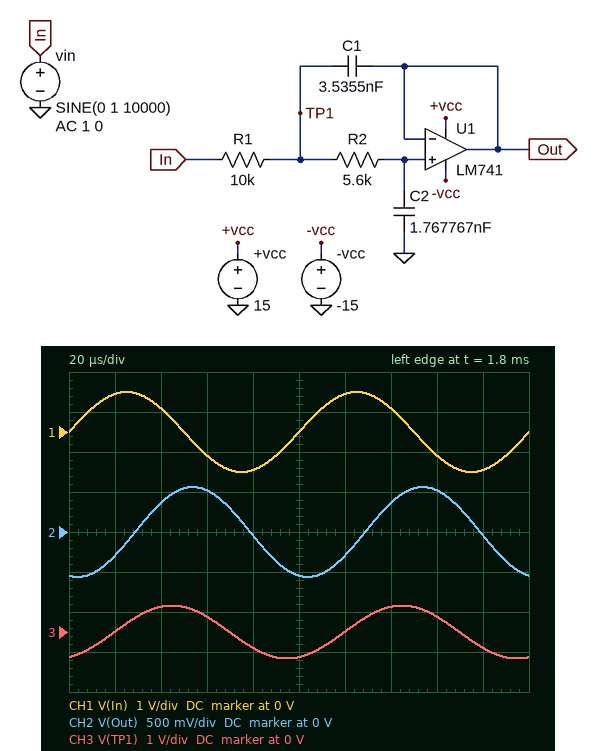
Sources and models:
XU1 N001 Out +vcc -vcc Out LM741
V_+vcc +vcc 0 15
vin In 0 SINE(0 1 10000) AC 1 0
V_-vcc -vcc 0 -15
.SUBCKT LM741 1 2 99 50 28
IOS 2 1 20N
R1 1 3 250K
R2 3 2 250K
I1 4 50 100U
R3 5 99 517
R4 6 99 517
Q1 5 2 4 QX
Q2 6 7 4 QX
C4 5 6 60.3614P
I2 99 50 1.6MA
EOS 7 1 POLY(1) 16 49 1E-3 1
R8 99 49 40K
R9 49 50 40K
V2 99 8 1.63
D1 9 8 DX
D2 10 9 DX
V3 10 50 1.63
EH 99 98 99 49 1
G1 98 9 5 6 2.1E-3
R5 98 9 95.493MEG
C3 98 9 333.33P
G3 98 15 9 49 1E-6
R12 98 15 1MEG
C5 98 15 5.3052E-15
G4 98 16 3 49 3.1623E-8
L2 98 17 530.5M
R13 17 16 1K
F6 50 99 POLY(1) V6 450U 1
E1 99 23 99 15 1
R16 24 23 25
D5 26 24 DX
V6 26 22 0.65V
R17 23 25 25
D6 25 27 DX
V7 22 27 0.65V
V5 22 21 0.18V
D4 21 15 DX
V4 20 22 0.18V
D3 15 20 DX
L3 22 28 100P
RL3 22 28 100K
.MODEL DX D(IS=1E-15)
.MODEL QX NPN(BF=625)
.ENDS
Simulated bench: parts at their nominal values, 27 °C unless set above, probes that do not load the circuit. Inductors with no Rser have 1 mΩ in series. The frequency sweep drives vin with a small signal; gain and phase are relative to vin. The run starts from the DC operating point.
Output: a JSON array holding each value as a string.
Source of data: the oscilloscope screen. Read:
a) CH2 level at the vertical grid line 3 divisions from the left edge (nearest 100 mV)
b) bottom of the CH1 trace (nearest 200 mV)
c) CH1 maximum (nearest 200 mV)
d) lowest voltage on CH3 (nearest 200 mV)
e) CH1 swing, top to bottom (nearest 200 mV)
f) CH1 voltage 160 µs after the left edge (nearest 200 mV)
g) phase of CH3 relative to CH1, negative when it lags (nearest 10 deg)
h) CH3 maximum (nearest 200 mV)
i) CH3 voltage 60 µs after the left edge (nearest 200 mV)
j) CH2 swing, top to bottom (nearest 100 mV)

["500 mV", "-1.0 V", "1.0 V", "-600 mV", "2.0 V", "-600 mV", "-70 deg", "600 mV", "400 mV", "1.1 V"]
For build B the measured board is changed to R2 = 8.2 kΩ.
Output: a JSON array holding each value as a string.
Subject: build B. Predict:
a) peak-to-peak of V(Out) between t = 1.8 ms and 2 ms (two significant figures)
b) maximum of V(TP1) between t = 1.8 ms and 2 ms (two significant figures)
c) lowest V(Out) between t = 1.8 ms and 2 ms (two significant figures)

["880 mV", "590 mV", "-440 mV"]
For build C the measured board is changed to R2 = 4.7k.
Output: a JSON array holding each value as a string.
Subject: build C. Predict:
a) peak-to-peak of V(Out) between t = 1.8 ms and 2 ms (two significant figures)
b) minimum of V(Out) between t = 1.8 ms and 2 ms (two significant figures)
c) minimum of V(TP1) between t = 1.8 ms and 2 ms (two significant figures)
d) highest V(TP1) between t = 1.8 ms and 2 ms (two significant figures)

["1.2 V", "-610 mV", "-690 mV", "690 mV"]
